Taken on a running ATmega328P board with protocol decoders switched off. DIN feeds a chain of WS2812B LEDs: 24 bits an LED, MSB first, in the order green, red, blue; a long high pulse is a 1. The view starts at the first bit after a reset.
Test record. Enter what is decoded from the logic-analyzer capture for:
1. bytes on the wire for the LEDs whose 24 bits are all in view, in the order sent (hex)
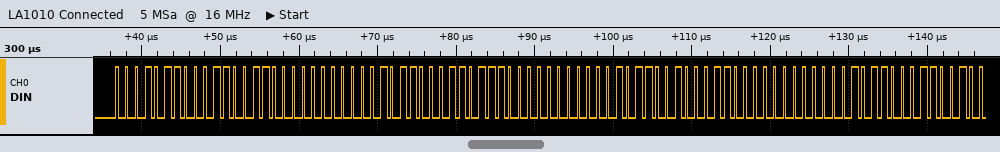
16 33 00 16 37 00 16 46 00
